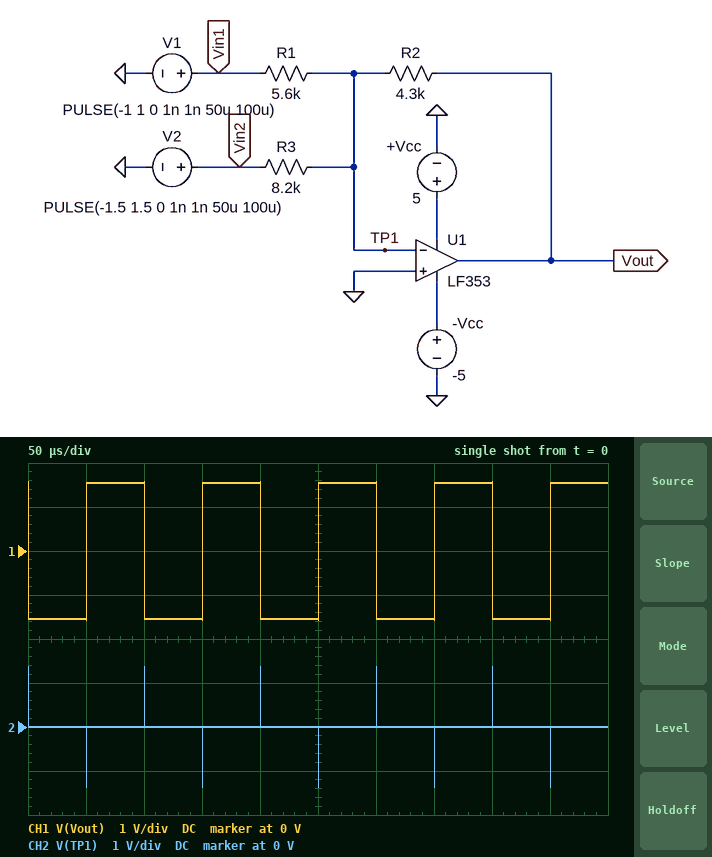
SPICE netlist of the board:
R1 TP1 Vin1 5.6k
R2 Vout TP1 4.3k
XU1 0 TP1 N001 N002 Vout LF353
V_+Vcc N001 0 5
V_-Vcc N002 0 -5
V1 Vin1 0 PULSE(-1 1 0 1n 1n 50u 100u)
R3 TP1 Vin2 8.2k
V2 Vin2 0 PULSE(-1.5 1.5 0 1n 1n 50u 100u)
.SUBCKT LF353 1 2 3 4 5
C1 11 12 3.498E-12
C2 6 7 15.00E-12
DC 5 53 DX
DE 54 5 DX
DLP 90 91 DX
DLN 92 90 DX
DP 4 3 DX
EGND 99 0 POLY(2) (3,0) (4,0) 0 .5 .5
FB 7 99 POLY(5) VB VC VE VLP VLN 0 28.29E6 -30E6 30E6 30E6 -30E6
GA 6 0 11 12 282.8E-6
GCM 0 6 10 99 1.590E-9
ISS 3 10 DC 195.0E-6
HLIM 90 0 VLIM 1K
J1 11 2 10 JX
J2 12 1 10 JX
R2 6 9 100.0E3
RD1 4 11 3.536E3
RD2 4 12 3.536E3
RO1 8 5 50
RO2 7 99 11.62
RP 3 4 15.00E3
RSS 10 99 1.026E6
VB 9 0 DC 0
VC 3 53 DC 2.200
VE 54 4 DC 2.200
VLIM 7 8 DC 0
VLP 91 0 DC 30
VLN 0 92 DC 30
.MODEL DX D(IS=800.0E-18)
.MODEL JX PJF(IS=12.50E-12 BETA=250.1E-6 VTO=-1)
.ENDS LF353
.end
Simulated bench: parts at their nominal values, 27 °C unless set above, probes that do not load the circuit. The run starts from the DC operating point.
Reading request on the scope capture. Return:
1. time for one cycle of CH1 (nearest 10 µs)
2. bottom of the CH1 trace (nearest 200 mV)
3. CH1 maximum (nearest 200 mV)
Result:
100 µs
-1.6 V
1.6 V
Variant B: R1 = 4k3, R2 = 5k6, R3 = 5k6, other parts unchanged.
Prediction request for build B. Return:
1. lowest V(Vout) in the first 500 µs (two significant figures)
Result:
-2.8 V
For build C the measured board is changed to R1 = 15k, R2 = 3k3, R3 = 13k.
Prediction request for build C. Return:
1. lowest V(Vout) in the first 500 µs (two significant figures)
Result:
-610 mV
